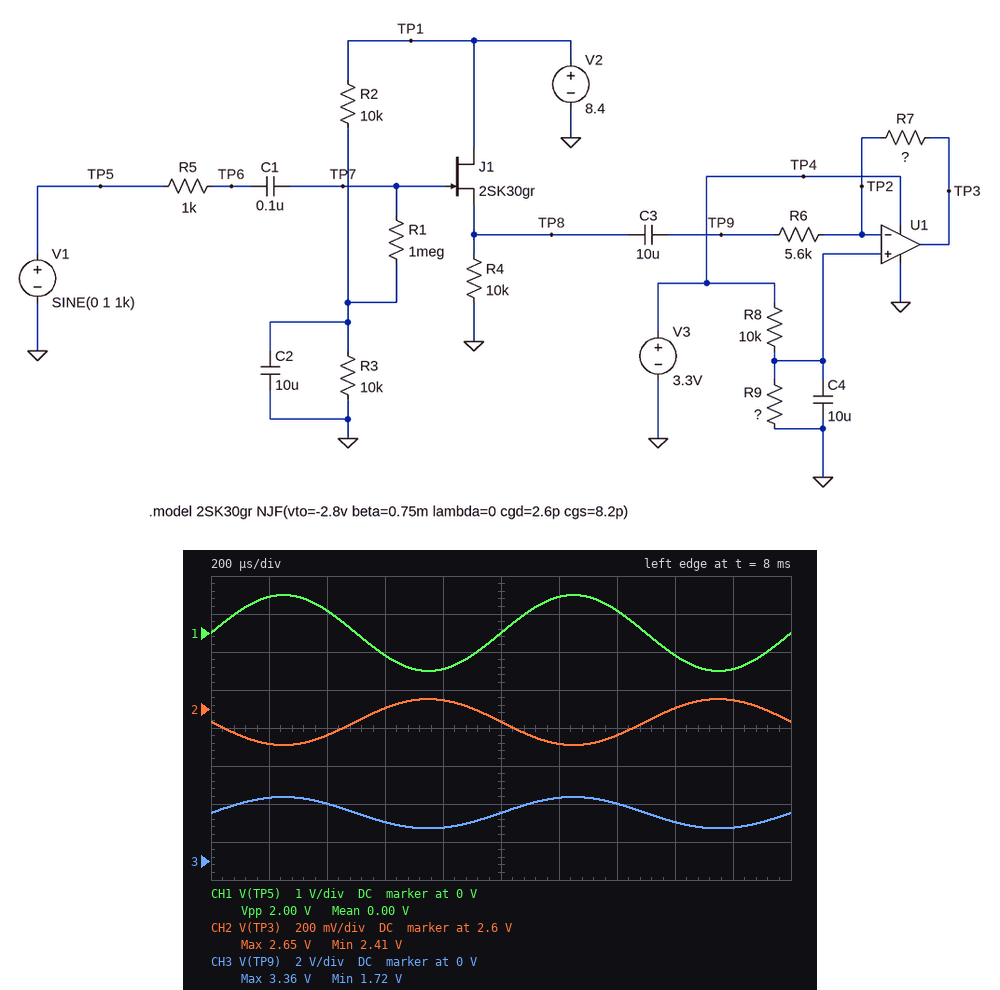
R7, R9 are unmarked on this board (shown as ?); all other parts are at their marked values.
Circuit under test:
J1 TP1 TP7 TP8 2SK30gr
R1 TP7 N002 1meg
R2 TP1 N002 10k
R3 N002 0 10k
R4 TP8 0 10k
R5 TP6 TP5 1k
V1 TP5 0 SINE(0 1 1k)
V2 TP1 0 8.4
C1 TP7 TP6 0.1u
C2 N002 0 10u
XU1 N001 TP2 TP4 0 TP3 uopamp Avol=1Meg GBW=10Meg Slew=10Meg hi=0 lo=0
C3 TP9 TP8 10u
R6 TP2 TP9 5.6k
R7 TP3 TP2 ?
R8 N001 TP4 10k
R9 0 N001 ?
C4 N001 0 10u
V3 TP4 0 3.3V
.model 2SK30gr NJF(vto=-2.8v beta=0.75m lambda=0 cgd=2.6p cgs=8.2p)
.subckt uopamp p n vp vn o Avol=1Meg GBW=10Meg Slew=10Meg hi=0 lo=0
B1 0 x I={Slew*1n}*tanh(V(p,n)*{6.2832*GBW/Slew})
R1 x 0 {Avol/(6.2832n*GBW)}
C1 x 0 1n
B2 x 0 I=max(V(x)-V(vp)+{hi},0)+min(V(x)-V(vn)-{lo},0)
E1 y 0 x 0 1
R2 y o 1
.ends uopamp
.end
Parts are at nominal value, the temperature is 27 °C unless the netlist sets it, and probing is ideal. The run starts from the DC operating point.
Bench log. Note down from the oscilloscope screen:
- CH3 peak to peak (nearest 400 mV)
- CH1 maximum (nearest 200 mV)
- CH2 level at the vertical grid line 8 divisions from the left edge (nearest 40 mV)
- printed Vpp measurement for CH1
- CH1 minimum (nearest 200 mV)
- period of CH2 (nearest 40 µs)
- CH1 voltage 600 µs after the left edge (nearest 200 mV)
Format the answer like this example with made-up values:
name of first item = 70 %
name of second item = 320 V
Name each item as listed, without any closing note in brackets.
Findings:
CH3 peak to peak = 1.6 V
CH1 maximum = 1.0 V
CH2 level at the vertical grid line 8 divisions from the left edge = 2.60 V
printed Vpp measurement for CH1 = 2.00 V
CH1 minimum = -1.0 V
period of CH2 = 1.00 ms
CH1 voltage 600 µs after the left edge = -600 mV
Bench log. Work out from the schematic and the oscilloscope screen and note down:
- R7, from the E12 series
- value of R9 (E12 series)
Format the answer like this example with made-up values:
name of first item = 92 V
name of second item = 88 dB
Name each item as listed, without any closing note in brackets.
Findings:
R7, from the E12 series = 820 Ω
value of R9 = 33 kΩ
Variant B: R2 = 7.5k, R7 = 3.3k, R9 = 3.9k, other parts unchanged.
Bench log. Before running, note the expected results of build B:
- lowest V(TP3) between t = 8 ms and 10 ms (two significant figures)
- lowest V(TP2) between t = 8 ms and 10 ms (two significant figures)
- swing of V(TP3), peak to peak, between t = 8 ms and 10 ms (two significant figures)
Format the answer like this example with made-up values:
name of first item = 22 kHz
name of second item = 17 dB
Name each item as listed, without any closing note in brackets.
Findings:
lowest V(TP3) between t = 8 ms and 10 ms = 440 mV
lowest V(TP2) between t = 8 ms and 10 ms = 930 mV
swing of V(TP3), peak to peak, between t = 8 ms and 10 ms = 970 mV
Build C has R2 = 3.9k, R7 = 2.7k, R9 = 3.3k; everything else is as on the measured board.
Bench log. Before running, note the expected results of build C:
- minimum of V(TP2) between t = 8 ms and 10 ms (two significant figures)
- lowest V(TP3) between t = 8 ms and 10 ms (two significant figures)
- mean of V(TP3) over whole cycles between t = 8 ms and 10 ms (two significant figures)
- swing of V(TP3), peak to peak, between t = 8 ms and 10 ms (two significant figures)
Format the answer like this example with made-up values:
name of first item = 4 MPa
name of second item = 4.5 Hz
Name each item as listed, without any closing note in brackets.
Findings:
minimum of V(TP2) between t = 8 ms and 10 ms = 820 mV
lowest V(TP3) between t = 8 ms and 10 ms = 660 mV
mean of V(TP3) over whole cycles between t = 8 ms and 10 ms = 870 mV
swing of V(TP3), peak to peak, between t = 8 ms and 10 ms = 520 mV
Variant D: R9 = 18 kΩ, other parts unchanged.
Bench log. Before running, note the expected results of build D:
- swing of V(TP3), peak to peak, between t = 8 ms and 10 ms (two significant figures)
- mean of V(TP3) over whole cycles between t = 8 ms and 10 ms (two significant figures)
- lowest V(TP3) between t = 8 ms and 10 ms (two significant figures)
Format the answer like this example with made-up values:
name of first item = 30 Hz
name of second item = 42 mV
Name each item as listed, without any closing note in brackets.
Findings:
swing of V(TP3), peak to peak, between t = 8 ms and 10 ms = 240 mV
mean of V(TP3) over whole cycles between t = 8 ms and 10 ms = 2.1 V
lowest V(TP3) between t = 8 ms and 10 ms = 2.0 V
